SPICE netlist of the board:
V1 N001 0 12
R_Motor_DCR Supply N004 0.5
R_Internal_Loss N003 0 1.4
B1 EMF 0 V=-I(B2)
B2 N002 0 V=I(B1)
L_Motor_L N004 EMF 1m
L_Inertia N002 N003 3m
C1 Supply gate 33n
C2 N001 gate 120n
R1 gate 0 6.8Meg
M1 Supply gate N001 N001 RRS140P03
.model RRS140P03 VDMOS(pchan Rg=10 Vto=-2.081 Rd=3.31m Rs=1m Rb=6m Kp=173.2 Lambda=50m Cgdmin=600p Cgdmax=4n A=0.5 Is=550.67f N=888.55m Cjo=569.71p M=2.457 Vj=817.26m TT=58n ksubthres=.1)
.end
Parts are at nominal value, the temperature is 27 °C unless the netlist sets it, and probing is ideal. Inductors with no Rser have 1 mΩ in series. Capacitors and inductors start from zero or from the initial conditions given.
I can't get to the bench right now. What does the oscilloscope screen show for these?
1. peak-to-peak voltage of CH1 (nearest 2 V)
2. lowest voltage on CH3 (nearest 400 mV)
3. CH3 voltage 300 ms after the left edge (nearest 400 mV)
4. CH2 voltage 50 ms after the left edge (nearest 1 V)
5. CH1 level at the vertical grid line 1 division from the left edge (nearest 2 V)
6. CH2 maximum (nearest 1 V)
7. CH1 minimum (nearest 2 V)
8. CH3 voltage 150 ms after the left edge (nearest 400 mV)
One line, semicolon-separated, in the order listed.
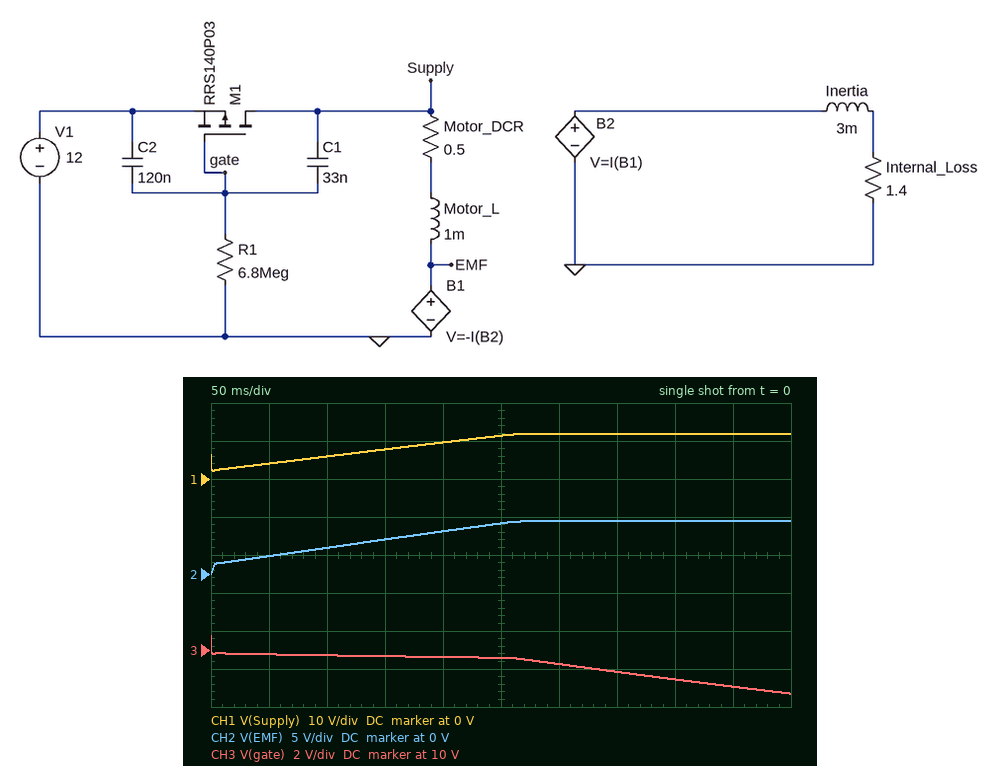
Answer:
10 V; 7.6 V; 9.2 V; 2 V; 4 V; 7 V; 2 V; 9.6 V
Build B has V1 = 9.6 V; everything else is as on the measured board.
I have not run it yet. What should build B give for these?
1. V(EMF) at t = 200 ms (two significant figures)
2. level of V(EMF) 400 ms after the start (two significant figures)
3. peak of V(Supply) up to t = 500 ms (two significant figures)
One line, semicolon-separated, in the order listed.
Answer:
3.3 V; 5.6 V; 9.5 V
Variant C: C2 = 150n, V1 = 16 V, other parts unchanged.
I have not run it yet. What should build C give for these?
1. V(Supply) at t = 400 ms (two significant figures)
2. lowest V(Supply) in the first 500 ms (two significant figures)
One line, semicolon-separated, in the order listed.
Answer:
16 V; 4.0 V
